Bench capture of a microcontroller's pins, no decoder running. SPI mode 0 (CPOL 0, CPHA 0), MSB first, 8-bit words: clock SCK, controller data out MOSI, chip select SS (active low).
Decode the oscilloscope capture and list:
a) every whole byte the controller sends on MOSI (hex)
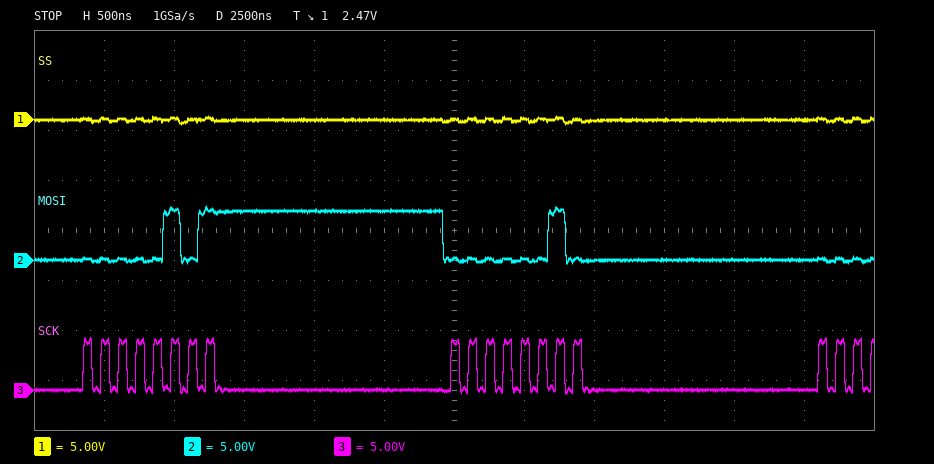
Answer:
0x05 0x02
